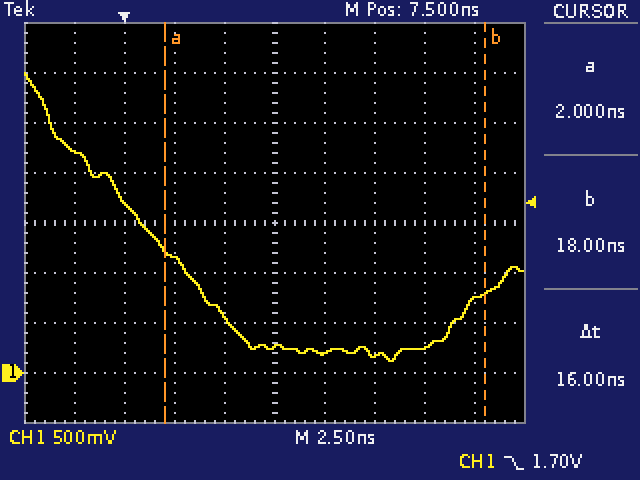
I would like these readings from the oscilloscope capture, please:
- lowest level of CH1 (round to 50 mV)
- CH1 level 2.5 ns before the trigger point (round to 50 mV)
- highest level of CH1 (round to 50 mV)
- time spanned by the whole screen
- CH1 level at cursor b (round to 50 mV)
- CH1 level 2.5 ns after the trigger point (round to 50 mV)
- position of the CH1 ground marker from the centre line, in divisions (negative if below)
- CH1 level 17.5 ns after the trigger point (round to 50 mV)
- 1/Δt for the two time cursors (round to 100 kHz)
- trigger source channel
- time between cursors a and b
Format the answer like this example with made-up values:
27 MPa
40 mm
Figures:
100 mV
2.20 V
3.00 V
25 ns
800 mV
1.15 V
-3.0 div
750 mV
62.5 MHz
CH1
16 ns
